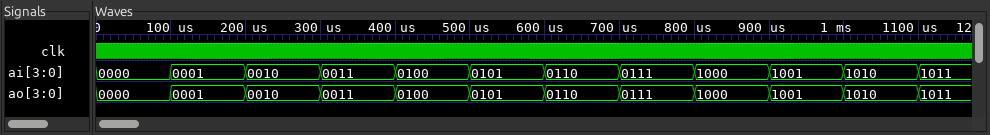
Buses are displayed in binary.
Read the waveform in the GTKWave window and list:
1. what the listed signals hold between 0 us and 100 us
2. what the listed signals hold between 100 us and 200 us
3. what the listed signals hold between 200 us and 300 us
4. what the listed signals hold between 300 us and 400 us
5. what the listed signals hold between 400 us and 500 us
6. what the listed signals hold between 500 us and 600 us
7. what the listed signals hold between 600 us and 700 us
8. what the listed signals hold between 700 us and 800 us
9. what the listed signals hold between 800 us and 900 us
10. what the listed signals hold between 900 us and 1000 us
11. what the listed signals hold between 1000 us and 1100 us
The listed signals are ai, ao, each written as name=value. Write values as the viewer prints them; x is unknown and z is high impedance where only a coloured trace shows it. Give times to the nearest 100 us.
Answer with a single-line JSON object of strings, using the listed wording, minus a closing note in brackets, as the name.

{"what the listed signals hold between 0 us and 100 us": "ai=0000, ao=0000", "what the listed signals hold between 100 us and 200 us": "ai=0001, ao=0001", "what the listed signals hold between 200 us and 300 us": "ai=0010, ao=0010", "what the listed signals hold between 300 us and 400 us": "ai=0011, ao=0011", "what the listed signals hold between 400 us and 500 us": "ai=0100, ao=0100", "what the listed signals hold between 500 us and 600 us": "ai=0101, ao=0101", "what the listed signals hold between 600 us and 700 us": "ai=0110, ao=0110", "what the listed signals hold between 700 us and 800 us": "ai=0111, ao=0111", "what the listed signals hold between 800 us and 900 us": "ai=1000, ao=1000", "what the listed signals hold between 900 us and 1000 us": "ai=1001, ao=1001", "what the listed signals hold between 1000 us and 1100 us": "ai=1010, ao=1010"}
